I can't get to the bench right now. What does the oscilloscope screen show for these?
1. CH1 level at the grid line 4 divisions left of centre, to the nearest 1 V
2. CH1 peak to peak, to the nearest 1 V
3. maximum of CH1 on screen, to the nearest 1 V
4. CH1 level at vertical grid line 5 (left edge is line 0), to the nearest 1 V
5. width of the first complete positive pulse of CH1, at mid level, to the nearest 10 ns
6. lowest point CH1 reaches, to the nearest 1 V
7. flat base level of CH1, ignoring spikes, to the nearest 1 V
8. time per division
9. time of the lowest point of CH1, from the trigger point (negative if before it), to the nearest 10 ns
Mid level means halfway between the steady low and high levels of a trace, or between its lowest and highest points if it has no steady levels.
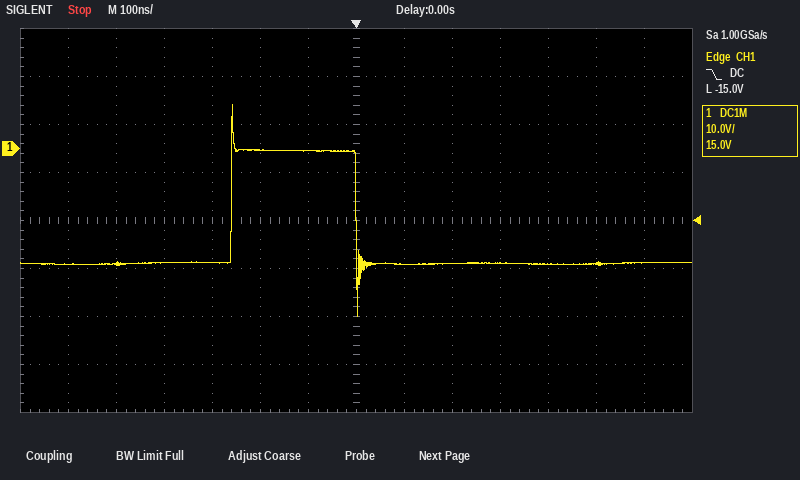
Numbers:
-24 V
44 V
9 V
0 V
260 ns
-35 V
-24 V
100 ns
0 ns
